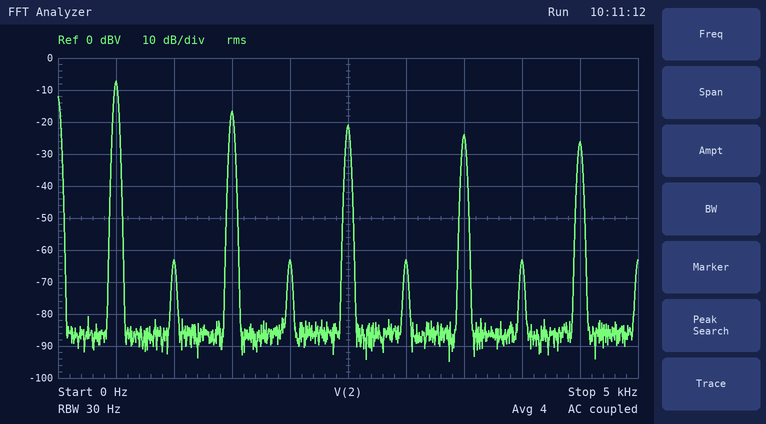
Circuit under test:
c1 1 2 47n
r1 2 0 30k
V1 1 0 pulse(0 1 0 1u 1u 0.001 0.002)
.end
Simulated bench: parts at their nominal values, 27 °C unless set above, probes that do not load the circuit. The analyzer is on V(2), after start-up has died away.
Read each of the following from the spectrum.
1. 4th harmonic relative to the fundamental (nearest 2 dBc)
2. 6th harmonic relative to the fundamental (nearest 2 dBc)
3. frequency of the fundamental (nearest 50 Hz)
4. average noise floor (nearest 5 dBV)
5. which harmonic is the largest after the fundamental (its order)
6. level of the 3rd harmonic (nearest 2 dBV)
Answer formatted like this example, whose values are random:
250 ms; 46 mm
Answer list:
-56 dBc; -56 dBc; 500 Hz; -85 dBV; 3; -16 dBV
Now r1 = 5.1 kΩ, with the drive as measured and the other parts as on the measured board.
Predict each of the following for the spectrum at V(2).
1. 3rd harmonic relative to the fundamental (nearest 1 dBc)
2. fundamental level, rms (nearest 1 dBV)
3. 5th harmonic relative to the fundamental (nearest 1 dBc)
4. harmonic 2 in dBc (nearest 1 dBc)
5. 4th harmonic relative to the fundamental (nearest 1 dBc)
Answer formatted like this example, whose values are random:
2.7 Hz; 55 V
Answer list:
-6 dBc; -11 dBV; -10 dBc; -53 dBc; -52 dBc
